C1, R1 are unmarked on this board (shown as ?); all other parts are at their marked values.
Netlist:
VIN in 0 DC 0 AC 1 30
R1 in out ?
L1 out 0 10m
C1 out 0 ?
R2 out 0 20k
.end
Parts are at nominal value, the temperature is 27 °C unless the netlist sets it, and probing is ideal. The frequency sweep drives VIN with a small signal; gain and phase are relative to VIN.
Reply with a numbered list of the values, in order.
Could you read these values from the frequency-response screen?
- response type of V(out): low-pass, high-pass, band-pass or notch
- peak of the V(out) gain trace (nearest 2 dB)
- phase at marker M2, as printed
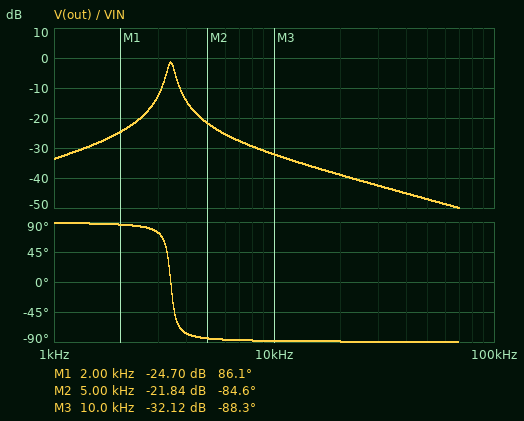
1. band-pass
2. -2 dB
3. -84.6 deg
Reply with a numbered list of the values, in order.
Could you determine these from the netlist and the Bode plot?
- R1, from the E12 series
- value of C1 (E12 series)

1. 3.3 kΩ
2. 220 nF
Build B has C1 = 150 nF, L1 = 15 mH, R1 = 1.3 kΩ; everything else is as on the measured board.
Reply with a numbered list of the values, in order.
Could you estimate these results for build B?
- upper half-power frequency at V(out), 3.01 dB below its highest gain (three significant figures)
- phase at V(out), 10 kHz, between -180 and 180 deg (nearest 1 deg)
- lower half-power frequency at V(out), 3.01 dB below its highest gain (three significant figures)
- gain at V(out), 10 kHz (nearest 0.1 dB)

1. 3.82 kHz
2. -84 deg
3. 2.95 kHz
4. -20.8 dB
